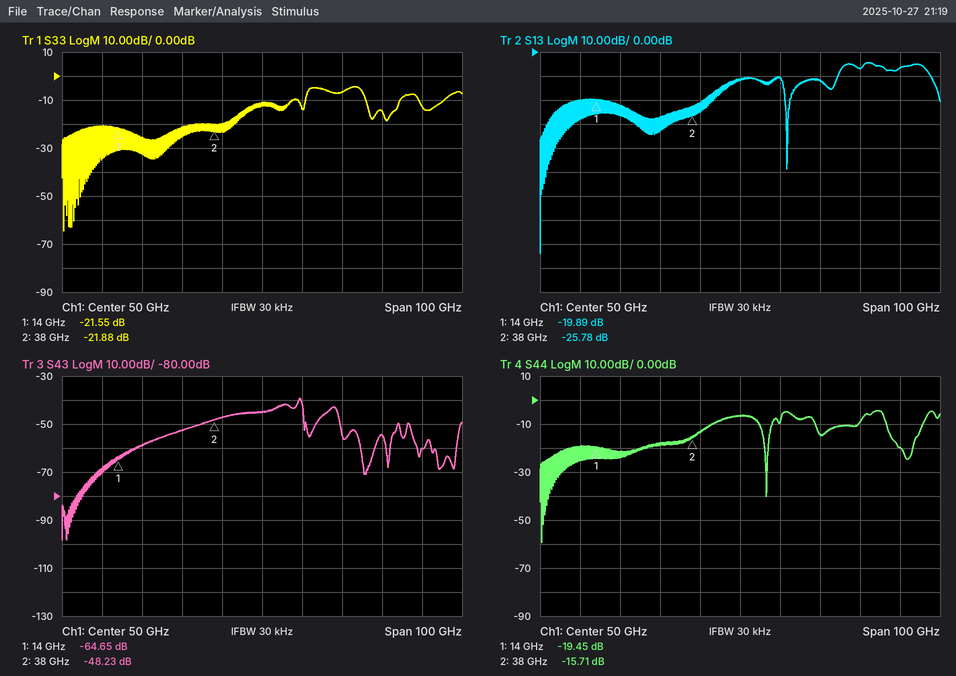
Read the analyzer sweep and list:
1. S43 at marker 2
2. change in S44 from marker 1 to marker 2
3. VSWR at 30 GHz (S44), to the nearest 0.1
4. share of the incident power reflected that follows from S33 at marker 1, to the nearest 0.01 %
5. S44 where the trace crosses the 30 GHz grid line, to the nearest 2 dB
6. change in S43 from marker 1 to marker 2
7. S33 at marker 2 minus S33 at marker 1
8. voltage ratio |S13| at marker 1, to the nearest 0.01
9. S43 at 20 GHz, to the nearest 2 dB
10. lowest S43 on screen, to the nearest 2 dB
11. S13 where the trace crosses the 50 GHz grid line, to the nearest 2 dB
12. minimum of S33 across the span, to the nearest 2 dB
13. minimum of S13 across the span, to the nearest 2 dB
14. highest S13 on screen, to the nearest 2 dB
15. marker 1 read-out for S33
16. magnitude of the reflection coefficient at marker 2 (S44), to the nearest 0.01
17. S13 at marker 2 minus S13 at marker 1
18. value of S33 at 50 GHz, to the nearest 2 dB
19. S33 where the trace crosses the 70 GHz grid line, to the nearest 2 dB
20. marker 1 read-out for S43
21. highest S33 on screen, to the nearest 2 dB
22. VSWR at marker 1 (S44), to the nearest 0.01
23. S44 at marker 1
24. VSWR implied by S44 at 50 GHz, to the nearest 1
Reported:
-48.23 dB
3.74 dB
1.3
0.70 %
-18 dB
16.42 dB
-0.33 dB
0.10
-58 dB
-98 dB
-12 dB
-64 dB
-84 dB
-4 dB
-21.55 dB
0.16
-5.89 dB
-12 dB
-6 dB
-64.65 dB
-4 dB
1.24
-19.45 dB
3
